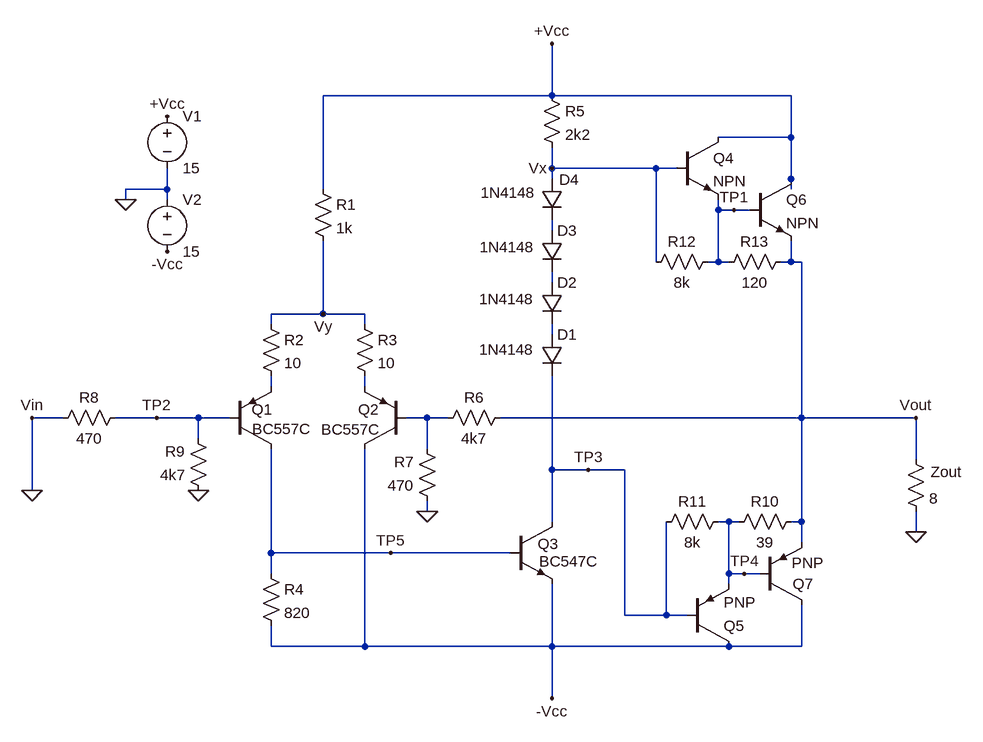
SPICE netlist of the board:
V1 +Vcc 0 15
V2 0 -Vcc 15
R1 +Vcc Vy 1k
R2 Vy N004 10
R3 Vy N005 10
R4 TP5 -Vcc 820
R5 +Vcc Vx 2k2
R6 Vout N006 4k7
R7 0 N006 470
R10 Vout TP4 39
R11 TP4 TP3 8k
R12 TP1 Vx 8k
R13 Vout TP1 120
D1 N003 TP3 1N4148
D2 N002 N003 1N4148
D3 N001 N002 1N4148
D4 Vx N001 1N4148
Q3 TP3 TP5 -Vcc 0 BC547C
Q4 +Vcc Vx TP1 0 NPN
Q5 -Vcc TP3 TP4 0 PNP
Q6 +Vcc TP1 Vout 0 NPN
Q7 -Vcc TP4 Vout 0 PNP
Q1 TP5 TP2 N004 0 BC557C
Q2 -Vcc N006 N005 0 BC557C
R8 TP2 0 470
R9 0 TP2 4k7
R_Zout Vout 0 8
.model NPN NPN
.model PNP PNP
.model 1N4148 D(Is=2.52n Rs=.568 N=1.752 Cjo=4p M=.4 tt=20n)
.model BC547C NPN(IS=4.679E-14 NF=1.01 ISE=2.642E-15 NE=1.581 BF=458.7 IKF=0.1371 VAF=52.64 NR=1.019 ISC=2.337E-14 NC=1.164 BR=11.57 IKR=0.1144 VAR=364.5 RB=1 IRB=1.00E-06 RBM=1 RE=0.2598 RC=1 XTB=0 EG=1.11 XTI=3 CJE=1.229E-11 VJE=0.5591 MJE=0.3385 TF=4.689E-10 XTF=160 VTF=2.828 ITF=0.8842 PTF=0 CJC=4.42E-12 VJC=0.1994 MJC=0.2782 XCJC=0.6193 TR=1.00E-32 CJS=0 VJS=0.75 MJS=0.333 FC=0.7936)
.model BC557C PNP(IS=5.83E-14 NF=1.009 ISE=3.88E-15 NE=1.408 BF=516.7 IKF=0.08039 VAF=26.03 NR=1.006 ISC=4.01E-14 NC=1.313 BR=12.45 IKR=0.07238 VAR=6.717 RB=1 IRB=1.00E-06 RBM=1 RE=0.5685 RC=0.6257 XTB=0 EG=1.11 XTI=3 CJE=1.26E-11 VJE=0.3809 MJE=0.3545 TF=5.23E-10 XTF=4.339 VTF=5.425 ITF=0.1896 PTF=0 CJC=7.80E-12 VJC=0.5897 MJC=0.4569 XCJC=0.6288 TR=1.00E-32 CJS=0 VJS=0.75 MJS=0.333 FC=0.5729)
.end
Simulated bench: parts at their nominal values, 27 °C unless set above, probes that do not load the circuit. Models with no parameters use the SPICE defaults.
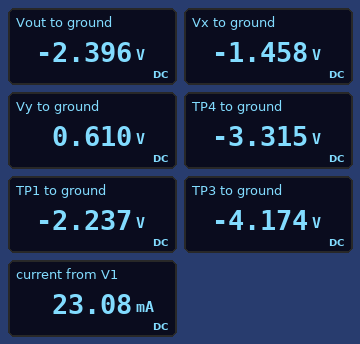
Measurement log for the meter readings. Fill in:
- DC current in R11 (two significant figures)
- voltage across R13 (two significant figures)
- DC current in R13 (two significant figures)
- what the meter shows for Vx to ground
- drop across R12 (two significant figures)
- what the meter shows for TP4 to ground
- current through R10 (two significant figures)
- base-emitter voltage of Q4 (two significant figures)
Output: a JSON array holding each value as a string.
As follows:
["110 µA", "160 mV", "1.3 mA", "-1.458 V", "780 mV", "-3.315 V", "24 mA", "780 mV"]
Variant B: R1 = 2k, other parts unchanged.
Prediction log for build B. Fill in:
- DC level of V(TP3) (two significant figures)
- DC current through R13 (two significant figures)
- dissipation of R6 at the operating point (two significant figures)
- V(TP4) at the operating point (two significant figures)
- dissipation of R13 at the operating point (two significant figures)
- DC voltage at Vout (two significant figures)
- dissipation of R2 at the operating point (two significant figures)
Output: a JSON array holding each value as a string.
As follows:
["-3.0 V", "1.4 mA", "290 µW", "-2.2 V", "220 µW", "-1.3 V", "6.9 µW"]
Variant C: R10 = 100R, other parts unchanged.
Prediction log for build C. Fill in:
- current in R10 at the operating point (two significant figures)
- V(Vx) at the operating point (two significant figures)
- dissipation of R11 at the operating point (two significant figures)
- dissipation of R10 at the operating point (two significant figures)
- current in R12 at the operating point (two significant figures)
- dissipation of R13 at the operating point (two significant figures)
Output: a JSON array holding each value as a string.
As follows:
["9.2 mA", "-1.4 V", "88 µW", "8.5 mW", "98 µA", "250 µW"]
